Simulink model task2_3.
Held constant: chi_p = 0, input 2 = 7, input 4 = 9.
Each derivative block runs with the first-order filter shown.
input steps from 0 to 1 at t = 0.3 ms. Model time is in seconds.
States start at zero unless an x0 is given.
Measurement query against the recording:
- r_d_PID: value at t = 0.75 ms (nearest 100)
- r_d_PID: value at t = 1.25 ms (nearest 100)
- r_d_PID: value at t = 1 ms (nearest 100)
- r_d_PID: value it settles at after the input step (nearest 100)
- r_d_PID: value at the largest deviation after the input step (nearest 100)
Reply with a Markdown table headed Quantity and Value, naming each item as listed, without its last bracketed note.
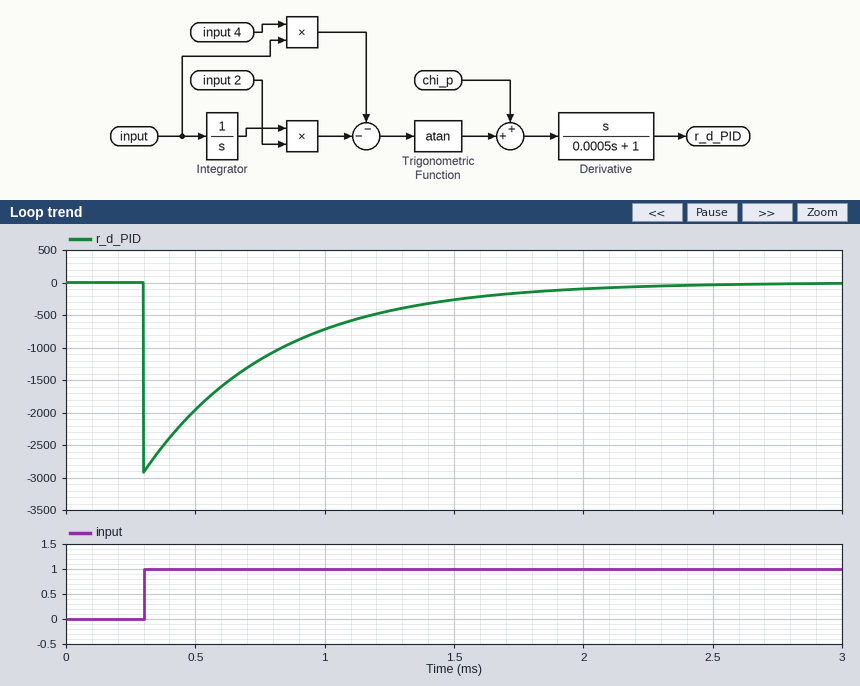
| Quantity | Value |
|---|---|
| r_d_PID: value at t = 0.75 ms | -1200 |
| r_d_PID: value at t = 1.25 ms | -400 |
| r_d_PID: value at t = 1 ms | -700 |
| r_d_PID: value it settles at after the input step | 0 |
| r_d_PID: value at the largest deviation after the input step | -2900 |
